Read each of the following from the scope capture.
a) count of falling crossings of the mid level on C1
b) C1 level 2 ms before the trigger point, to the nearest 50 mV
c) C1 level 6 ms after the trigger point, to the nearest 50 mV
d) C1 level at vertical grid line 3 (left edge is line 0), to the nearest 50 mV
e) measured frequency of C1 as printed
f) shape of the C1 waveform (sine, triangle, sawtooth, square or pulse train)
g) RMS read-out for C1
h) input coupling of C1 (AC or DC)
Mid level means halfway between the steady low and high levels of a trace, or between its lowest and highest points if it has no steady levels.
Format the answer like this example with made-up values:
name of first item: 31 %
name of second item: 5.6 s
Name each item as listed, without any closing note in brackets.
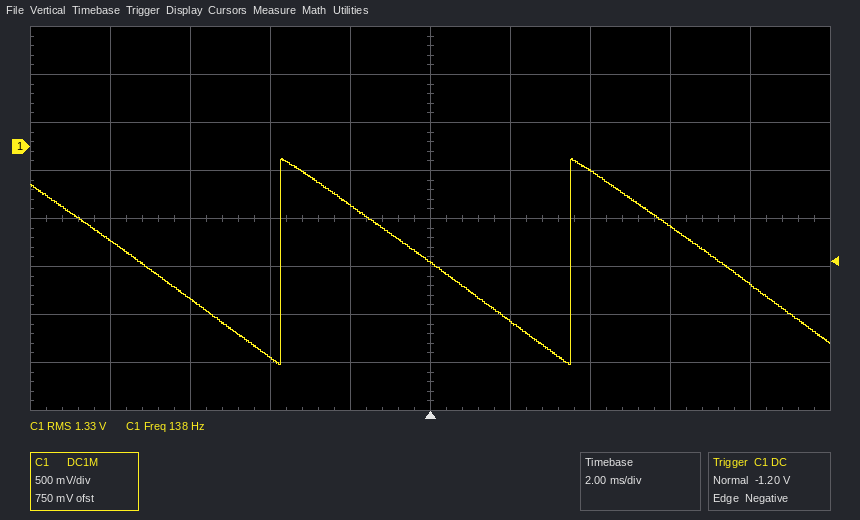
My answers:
count of falling crossings of the mid level on C1: 3
C1 level 2 ms before the trigger point, to the nearest 50 mV: -600 mV
C1 level 6 ms after the trigger point, to the nearest 50 mV: -850 mV
C1 level at vertical grid line 3 (left edge is line 0), to the nearest 50 mV: -2.20 V
measured frequency of C1 as printed: 138 Hz
shape of the C1 waveform: sawtooth
RMS read-out for C1: 1.33 V
input coupling of C1: DC
